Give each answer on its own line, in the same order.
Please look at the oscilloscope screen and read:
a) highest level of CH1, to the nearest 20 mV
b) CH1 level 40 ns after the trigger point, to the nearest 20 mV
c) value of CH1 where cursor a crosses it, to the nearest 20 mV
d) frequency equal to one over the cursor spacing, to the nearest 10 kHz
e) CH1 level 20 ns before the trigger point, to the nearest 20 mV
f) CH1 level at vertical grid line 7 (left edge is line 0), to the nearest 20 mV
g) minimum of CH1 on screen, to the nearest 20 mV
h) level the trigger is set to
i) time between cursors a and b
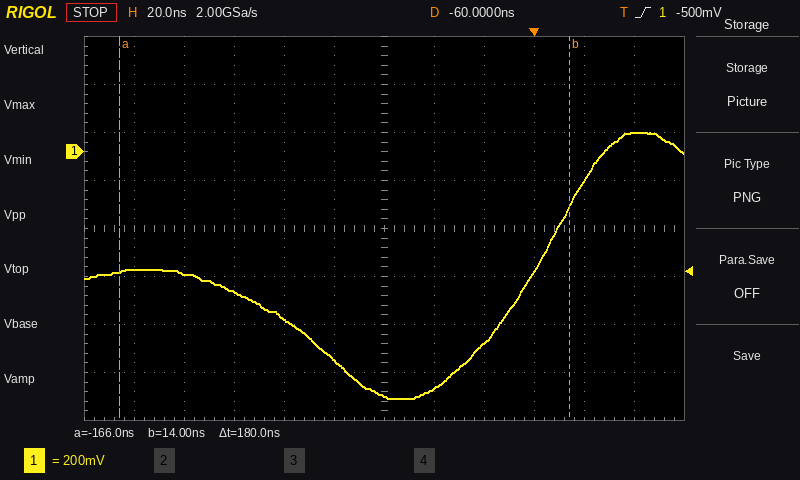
80 mV
80 mV
-500 mV
5.56 MHz
-800 mV
-980 mV
-1.02 V
-500 mV
180 ns
